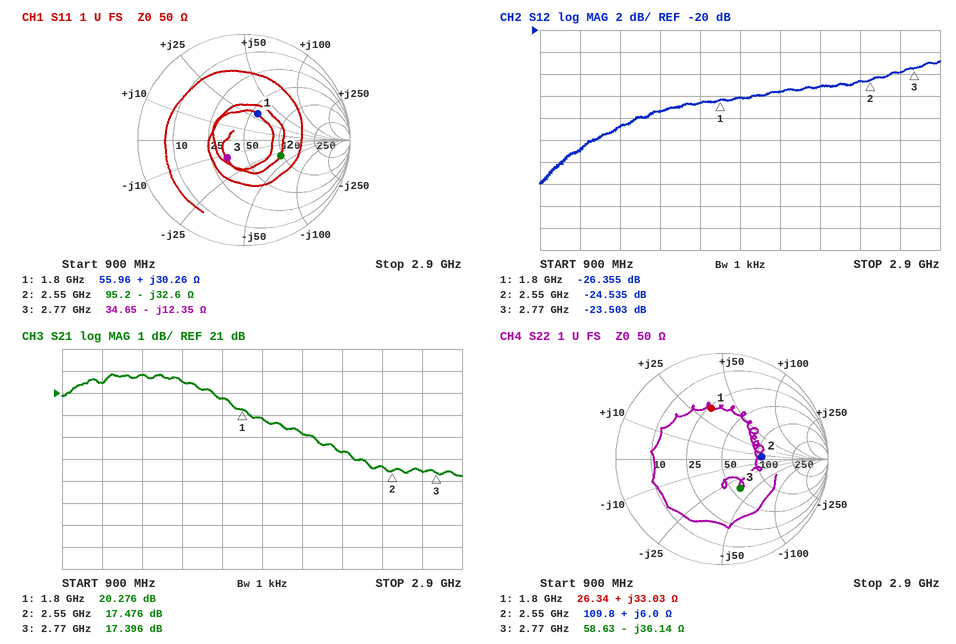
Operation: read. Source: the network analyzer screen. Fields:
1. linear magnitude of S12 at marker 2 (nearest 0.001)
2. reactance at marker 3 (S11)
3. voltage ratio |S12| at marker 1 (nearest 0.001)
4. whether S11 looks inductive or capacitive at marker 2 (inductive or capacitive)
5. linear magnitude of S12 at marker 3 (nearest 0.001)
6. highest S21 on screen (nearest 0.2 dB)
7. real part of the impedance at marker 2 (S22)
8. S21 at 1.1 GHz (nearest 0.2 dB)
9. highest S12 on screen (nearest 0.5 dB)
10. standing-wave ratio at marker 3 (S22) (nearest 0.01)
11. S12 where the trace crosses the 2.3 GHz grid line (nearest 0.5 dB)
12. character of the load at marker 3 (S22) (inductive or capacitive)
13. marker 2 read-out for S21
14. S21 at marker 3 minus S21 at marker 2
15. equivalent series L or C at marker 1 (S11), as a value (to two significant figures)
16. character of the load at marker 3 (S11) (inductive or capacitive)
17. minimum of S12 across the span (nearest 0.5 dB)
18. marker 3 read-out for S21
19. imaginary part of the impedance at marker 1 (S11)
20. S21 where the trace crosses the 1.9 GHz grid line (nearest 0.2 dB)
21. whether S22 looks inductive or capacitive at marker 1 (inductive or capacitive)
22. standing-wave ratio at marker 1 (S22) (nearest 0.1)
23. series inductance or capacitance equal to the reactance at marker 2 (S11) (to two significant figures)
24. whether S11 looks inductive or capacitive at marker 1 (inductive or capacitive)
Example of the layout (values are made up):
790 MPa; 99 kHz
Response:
0.059; -12.35 Ω; 0.048; capacitive; 0.067; 21.8 dB; 109.8 Ω; 21.4 dB; -23.0 dB; 1.96; -25.0 dB; capacitive; 17.476 dB; -0.080 dB; 2.7 nH; capacitive; -34.0 dB; 17.396 dB; +30.26 Ω; 19.8 dB; inductive; 2.9; 1.9 pF; inductive
